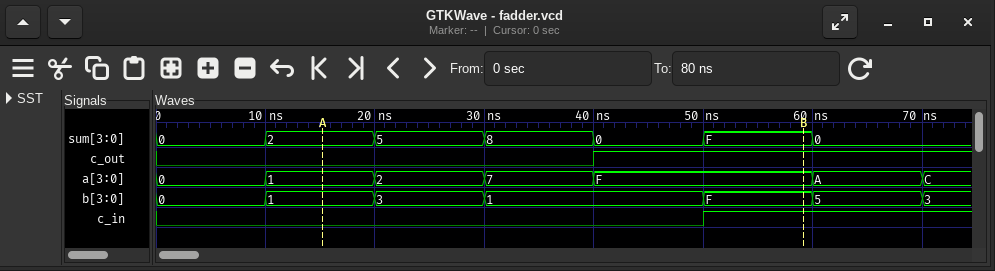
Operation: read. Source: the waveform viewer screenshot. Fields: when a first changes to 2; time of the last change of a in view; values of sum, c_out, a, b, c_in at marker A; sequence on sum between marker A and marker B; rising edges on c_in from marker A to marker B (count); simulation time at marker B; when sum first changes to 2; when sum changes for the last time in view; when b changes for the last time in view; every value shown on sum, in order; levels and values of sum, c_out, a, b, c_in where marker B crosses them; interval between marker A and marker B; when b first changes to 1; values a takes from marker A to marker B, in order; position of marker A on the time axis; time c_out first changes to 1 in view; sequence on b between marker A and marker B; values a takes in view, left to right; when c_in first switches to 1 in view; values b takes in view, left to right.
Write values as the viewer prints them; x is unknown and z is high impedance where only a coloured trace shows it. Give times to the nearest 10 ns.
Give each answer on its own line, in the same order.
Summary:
20 ns
70 ns
sum=2, c_out=0, a=1, b=1, c_in=0
2, 5, 8, 0, F
1
60 ns
10 ns
60 ns
70 ns
0, 2, 5, 8, 0, F, 0
sum=F, c_out=1, a=F, b=F, c_in=1
40 ns
10 ns
1, 2, 7, F
20 ns
40 ns
1, 3, 1, F
0, 1, 2, 7, F, A, C
50 ns
0, 1, 3, 1, F, 5, 3
